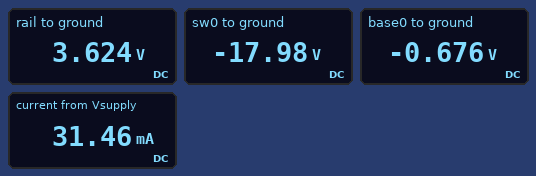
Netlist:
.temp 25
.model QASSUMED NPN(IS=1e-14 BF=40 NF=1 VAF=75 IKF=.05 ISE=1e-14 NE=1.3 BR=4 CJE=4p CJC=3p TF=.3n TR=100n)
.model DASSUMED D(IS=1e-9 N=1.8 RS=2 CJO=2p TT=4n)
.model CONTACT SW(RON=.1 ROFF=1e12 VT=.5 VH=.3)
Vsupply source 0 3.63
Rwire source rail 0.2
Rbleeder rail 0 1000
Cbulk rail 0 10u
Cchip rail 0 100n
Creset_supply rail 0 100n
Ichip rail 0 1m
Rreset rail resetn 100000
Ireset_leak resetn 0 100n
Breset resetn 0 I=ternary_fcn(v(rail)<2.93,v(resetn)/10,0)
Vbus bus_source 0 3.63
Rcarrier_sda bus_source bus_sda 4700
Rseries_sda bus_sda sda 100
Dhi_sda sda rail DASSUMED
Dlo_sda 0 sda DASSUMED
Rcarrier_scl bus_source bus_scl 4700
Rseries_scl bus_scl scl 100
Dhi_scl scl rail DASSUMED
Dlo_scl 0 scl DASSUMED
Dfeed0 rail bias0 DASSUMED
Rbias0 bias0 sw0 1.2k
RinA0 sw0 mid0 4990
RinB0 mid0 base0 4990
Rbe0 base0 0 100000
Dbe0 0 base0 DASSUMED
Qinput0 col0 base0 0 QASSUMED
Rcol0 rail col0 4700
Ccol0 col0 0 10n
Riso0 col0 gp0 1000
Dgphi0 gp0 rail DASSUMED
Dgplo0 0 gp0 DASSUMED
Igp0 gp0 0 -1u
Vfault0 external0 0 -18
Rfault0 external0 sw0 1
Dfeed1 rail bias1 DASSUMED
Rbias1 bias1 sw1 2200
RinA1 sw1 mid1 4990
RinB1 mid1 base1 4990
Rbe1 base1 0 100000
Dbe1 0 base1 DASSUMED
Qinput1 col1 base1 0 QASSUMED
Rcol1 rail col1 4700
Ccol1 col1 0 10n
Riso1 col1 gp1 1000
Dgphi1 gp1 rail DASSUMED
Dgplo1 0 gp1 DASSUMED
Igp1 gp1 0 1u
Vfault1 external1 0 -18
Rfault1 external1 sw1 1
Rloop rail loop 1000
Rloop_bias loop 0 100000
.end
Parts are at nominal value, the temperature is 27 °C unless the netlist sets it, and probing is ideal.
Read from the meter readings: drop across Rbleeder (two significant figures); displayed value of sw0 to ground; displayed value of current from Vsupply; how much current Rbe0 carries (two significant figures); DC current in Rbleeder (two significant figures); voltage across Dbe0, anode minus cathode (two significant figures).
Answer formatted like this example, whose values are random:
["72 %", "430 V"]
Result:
["3.6 V", "-17.98 V", "31.46 mA", "6.8 µA", "3.6 mA", "680 mV"]
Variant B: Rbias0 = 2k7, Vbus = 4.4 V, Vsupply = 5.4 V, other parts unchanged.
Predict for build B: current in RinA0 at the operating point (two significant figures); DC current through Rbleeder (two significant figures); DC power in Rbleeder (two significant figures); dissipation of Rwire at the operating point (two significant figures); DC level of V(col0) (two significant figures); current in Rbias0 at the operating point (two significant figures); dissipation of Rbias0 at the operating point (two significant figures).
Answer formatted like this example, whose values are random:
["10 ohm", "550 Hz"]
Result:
["1.7 mA", "5.4 mA", "29 mW", "130 µW", "5.4 V", "8.4 mA", "190 mW"]
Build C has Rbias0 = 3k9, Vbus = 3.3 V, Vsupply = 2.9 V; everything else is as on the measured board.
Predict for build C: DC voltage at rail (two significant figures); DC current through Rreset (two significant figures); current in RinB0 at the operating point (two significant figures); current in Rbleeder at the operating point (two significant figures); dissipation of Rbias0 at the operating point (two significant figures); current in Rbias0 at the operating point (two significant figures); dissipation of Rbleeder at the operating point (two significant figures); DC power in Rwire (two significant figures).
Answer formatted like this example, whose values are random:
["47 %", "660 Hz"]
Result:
["2.9 V", "29 µA", "1.7 mA", "2.9 mA", "100 mW", "5.2 mA", "8.4 mW", "67 µW"]
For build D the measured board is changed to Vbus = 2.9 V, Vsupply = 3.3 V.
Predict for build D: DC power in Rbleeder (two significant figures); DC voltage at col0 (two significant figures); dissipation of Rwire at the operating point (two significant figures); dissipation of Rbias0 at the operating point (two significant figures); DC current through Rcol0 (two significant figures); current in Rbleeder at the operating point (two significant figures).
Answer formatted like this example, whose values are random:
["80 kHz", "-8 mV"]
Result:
["11 mW", "3.3 V", "190 µW", "350 mW", "1.0 µA", "3.3 mA"]
